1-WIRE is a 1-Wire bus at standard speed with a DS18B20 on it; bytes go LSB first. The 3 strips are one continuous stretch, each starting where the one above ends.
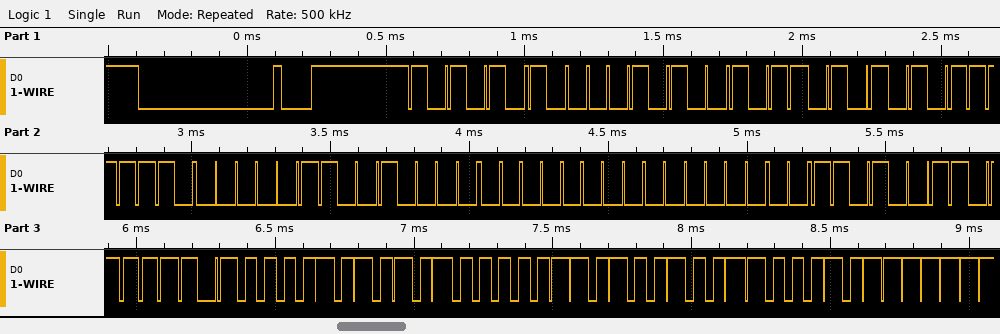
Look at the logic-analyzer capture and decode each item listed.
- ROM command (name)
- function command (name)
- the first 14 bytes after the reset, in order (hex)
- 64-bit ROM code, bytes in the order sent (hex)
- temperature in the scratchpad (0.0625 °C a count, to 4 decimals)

Match ROM
Read Scratchpad
55 28 AD FA 81 09 00 00 CB BE 50 05 4B 46
28 AD FA 81 09 00 00 CB
85.0000 °C
